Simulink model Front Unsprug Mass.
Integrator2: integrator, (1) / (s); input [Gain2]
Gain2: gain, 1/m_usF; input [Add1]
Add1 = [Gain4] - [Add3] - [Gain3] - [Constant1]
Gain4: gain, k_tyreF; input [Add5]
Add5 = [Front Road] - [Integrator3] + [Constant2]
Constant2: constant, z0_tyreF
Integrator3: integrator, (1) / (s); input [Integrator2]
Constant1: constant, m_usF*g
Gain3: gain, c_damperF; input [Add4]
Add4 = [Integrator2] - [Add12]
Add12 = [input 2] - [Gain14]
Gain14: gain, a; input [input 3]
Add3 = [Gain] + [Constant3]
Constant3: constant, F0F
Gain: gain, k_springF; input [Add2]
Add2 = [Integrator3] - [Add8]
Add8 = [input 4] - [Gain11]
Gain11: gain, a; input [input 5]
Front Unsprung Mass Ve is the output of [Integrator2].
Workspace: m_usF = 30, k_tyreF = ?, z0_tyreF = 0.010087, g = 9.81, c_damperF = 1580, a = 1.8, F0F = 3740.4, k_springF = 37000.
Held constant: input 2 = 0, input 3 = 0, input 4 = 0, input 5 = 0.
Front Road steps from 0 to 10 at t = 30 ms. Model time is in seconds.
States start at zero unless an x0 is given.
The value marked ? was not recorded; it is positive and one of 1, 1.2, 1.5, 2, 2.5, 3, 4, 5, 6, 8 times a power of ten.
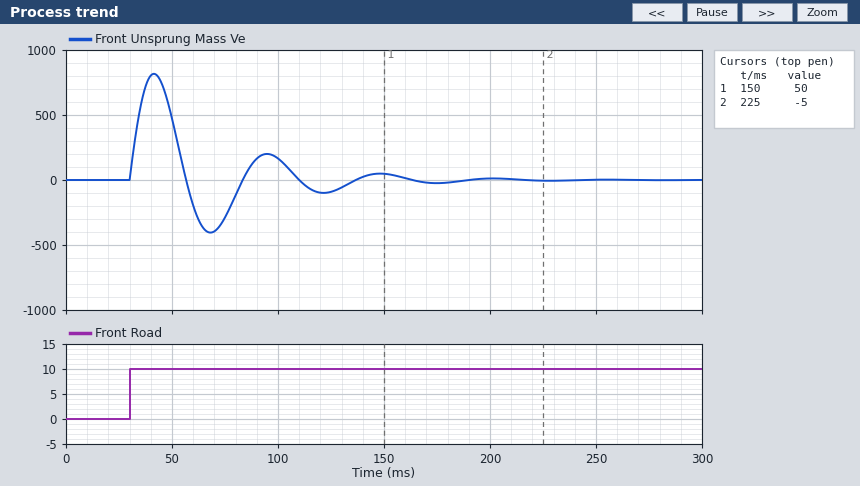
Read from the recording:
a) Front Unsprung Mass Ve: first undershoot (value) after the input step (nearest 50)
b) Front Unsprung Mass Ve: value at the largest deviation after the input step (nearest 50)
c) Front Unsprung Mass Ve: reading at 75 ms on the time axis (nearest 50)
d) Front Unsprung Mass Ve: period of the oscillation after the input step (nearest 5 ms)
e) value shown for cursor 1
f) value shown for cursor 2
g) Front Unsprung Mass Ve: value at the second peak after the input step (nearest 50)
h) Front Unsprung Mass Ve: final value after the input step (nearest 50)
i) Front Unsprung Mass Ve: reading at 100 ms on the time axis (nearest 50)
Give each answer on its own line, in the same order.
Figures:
-400
800
-300
55 ms
50
-5
200
0
150
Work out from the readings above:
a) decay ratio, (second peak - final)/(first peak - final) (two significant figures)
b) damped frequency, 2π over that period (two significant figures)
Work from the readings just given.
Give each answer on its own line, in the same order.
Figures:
0.25
0.11 rad/ms
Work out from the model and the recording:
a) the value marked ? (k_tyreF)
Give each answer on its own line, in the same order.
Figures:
400000
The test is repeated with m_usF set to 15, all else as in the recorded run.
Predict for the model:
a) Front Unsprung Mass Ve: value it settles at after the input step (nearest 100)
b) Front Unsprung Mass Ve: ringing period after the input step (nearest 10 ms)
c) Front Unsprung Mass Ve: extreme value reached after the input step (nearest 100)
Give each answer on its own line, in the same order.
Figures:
0
40 ms
1000
